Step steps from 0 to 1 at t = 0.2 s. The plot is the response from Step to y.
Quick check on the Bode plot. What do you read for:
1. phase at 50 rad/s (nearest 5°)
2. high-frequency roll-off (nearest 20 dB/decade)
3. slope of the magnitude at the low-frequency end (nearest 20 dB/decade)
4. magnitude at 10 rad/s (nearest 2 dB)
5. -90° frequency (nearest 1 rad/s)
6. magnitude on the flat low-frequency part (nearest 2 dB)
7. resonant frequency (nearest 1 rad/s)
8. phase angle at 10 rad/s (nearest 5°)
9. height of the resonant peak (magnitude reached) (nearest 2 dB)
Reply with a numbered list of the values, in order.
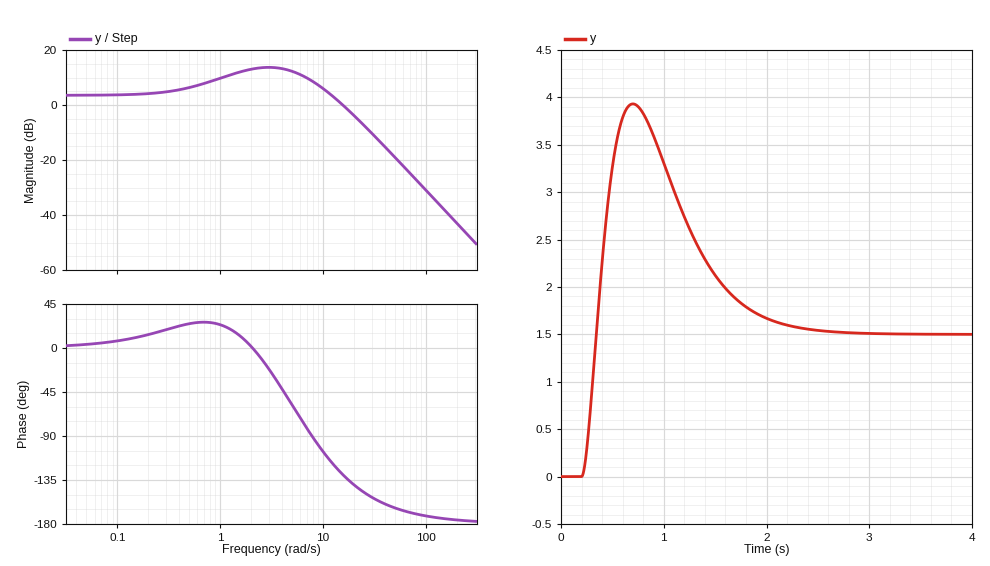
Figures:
1. -165°
2. -40 dB/decade
3. 0 dB/decade
4. 6 dB
5. 8 rad/s
6. 4 dB
7. 3 rad/s
8. -105°
9. 14 dB
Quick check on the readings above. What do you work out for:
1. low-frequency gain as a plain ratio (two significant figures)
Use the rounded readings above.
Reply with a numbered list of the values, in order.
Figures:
1. 1.6
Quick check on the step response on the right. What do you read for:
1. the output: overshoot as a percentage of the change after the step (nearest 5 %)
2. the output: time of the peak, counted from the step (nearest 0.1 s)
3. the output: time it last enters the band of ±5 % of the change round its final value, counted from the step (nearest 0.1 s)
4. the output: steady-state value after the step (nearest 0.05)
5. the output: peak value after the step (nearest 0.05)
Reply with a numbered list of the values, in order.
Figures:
1. 160 %
2. 0.5 s
3. 2.1 s
4. 1.50
5. 3.95
